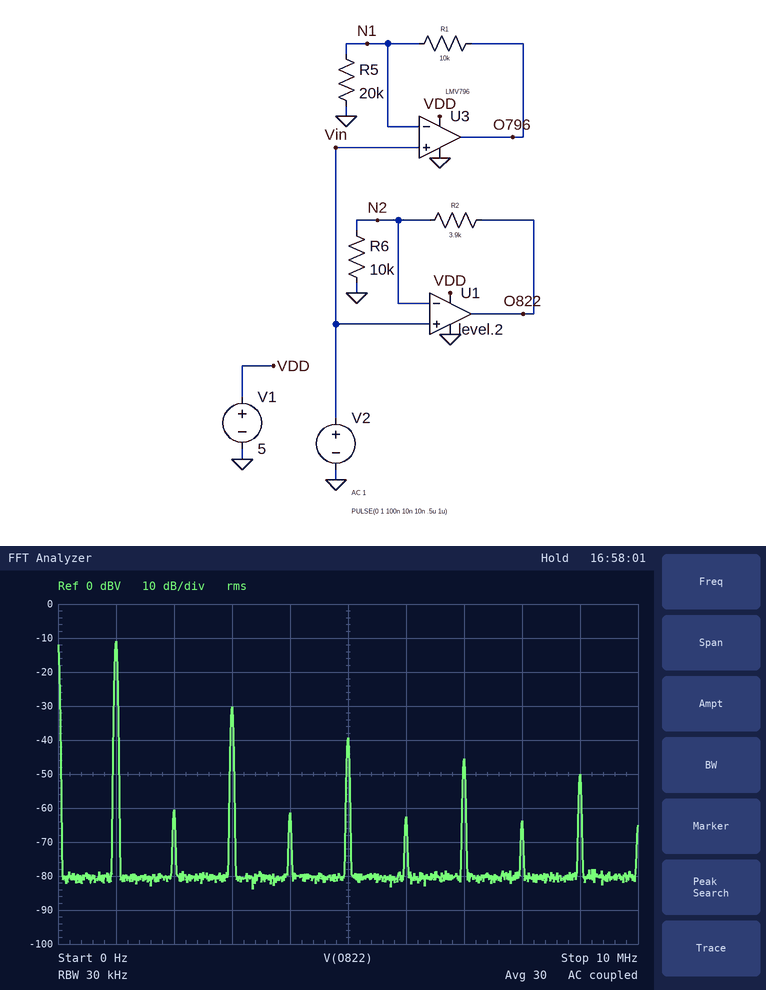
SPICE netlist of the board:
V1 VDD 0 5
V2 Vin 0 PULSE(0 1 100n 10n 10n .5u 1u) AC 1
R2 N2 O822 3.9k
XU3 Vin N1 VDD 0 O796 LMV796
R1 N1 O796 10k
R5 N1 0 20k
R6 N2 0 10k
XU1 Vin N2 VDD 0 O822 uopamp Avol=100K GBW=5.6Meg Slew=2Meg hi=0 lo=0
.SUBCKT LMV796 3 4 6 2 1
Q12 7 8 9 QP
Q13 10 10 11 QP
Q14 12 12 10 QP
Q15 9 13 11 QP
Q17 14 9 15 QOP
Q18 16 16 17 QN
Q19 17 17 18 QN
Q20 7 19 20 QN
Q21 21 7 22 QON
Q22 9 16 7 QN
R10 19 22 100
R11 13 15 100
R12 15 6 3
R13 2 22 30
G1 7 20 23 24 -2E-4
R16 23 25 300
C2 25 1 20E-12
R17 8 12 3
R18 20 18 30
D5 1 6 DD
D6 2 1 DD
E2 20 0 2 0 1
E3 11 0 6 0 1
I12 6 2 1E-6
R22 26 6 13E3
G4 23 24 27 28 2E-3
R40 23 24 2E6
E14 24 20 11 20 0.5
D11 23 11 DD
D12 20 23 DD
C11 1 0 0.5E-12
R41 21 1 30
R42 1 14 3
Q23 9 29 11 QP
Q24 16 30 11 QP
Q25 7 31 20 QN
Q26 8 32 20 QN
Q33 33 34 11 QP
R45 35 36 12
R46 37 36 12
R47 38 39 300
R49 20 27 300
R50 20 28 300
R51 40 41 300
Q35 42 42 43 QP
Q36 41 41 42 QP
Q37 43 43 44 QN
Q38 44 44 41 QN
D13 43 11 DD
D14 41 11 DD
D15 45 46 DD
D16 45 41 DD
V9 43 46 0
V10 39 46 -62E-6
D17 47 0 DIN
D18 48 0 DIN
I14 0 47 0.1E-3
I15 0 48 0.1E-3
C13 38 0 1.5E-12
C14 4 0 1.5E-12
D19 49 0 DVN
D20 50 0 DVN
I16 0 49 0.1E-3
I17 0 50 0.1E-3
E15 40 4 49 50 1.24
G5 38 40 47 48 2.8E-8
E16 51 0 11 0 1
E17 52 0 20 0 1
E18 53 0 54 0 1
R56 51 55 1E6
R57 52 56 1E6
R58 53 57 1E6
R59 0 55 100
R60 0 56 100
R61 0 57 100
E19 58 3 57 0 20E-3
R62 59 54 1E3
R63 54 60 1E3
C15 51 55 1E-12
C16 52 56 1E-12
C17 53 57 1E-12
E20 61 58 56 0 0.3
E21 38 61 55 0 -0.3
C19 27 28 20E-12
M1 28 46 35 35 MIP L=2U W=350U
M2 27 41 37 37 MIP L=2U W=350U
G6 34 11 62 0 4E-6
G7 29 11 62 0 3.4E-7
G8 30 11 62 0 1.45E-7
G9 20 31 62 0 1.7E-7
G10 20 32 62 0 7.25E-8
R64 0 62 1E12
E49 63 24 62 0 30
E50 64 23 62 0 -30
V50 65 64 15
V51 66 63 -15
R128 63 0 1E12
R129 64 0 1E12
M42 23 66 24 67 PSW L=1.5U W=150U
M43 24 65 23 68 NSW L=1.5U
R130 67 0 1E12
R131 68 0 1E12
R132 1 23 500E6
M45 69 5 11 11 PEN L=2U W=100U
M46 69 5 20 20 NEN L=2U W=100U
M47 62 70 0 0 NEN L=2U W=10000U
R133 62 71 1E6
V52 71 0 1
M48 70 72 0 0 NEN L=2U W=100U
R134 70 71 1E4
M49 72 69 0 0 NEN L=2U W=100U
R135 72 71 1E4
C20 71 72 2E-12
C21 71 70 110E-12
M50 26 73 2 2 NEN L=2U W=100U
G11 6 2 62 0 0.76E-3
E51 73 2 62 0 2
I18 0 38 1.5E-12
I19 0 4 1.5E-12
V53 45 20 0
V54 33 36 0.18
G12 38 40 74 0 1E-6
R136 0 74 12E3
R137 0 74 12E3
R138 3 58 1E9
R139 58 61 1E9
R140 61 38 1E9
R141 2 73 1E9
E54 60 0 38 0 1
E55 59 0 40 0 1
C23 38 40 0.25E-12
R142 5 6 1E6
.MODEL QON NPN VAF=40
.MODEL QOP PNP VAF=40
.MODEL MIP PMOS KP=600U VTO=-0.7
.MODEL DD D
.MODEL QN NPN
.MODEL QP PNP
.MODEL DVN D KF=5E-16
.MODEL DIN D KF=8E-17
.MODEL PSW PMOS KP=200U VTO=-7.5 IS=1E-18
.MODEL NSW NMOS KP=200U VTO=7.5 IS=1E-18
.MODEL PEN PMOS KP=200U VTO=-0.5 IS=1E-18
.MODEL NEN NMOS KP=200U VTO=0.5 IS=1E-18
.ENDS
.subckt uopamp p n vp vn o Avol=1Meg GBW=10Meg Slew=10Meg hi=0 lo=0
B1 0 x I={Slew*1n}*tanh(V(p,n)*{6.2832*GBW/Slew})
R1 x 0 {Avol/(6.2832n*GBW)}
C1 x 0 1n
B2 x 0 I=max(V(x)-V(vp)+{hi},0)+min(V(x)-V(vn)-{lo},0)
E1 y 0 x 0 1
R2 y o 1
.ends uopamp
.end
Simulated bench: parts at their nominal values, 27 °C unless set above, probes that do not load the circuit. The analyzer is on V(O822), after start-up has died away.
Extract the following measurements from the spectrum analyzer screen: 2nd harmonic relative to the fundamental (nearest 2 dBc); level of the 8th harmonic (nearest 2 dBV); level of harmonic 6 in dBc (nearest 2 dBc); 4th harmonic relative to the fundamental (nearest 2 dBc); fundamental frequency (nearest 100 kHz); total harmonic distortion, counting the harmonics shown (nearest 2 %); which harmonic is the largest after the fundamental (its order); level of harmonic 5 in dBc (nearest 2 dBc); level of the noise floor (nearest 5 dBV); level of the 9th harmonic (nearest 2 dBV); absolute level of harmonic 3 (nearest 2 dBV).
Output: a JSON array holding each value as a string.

["-50 dBc", "-64 dBV", "-52 dBc", "-50 dBc", "1.0 MHz", "12 %", "3", "-28 dBc", "-80 dBV", "-50 dBV", "-30 dBV"]
